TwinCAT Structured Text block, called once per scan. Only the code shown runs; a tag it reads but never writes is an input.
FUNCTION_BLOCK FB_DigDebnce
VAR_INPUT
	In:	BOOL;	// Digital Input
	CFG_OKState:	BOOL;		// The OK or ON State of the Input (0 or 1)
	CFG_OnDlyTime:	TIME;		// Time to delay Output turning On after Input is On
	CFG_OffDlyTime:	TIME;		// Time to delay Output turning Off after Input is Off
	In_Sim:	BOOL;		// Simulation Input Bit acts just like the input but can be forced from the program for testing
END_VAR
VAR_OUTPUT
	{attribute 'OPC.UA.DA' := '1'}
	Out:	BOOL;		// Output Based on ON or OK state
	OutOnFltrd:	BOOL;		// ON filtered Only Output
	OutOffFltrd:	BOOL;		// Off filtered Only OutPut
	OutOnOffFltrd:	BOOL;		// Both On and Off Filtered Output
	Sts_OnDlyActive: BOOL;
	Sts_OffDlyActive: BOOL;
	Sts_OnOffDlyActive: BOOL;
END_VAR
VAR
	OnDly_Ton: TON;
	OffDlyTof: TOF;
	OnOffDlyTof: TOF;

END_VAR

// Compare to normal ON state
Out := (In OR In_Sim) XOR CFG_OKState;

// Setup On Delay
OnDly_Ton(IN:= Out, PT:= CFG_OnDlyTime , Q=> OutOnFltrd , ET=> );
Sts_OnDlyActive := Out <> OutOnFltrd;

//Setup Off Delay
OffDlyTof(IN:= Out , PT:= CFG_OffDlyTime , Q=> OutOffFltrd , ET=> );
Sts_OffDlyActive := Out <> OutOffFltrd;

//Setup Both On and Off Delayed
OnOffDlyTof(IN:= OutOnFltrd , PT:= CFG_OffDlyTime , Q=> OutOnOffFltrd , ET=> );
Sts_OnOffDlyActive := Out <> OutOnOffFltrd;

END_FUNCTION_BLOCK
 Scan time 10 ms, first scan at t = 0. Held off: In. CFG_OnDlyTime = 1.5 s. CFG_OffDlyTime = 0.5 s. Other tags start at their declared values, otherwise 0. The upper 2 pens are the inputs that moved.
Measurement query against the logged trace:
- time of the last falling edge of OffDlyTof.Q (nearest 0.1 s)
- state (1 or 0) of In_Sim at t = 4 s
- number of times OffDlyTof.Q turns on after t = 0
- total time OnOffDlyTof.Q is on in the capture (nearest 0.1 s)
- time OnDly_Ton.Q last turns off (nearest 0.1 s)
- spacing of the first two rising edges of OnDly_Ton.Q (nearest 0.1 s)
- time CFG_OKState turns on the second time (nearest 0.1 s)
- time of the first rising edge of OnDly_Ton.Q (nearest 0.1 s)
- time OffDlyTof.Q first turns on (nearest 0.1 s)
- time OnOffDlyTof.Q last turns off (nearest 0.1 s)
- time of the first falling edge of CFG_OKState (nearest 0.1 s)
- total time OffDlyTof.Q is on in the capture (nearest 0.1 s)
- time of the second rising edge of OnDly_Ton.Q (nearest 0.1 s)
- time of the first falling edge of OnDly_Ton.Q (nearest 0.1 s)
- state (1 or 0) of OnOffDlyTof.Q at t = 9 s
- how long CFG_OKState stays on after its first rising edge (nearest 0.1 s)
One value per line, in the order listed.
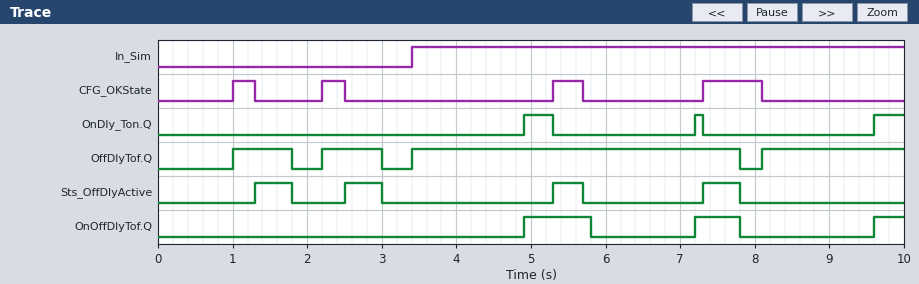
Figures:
7.8 s
1
4
1.9 s
7.3 s
2.3 s
2.2 s
4.9 s
1.0 s
7.8 s
1.3 s
7.9 s
7.2 s
5.3 s
0
0.3 s
